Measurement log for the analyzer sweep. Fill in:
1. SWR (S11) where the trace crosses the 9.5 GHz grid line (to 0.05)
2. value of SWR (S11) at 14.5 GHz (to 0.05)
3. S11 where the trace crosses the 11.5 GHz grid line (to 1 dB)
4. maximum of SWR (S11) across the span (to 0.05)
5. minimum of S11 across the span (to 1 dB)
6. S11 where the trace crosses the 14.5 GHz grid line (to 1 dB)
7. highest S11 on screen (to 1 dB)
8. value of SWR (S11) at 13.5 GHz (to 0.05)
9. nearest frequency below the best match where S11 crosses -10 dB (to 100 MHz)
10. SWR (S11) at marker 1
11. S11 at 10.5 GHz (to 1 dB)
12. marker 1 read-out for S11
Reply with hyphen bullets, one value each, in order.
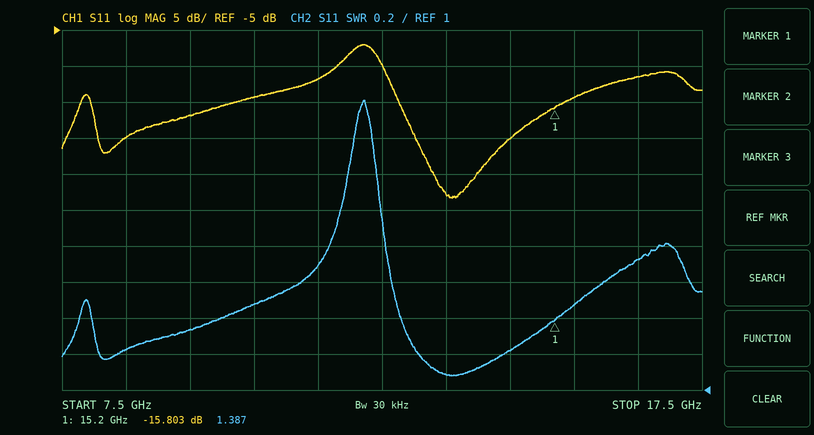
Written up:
- 1.35
- 1.20
- -12 dB
- 2.60
- -28 dB
- -20 dB
- -7 dB
- 1.10
- 12.5 GHz
- 1.387
- -14 dB
- -15.803 dB
